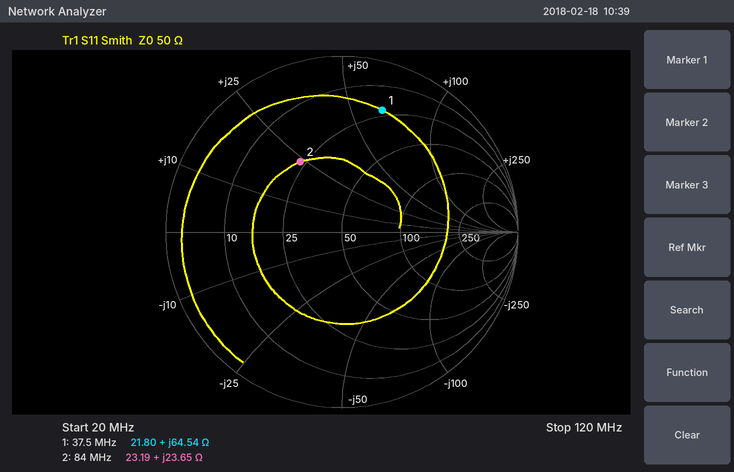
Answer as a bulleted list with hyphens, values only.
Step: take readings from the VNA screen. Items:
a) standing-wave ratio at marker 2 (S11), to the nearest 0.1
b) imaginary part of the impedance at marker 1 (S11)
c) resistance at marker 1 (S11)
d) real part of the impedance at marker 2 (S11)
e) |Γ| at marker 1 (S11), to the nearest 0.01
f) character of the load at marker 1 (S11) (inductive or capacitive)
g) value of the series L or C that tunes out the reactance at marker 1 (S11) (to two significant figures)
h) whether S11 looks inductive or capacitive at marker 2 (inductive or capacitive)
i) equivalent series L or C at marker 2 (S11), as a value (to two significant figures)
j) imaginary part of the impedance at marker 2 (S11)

- 2.7
- +64.54 Ω
- 21.80 Ω
- 23.19 Ω
- 0.73
- inductive
- 66 pF
- inductive
- 45 nH
- +23.65 Ω
